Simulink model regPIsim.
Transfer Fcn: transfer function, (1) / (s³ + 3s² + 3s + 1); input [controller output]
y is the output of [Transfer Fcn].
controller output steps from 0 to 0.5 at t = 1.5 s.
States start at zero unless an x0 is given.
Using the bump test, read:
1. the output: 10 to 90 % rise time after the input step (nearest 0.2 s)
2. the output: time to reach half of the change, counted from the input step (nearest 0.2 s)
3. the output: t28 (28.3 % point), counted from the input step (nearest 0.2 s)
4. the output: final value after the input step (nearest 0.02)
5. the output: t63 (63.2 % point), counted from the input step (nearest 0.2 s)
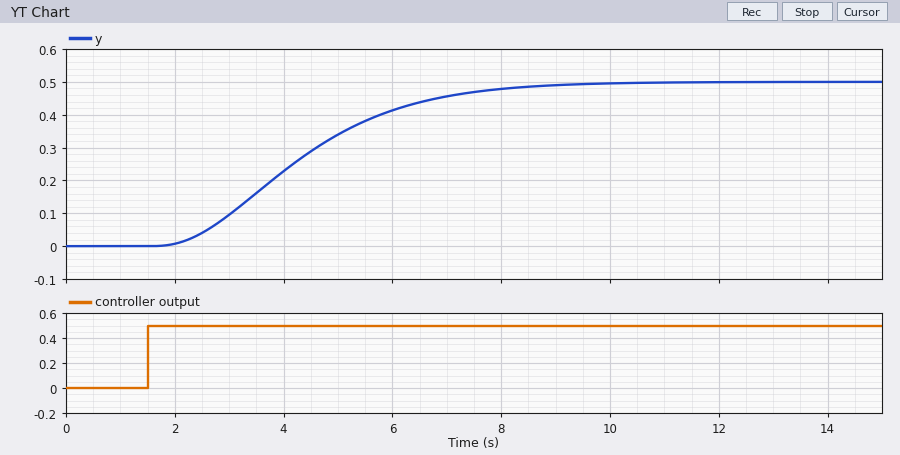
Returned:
4.2 s
2.6 s
1.8 s
0.50
3.2 s
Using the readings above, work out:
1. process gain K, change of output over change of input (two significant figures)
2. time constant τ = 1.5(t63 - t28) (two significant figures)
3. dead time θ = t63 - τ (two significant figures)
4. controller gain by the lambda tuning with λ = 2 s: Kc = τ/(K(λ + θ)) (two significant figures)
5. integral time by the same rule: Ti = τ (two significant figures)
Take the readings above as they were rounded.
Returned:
1.0
2.1 s
1.1 s
0.68
2.1 s
